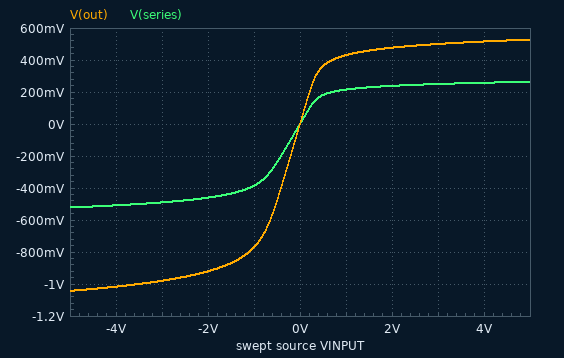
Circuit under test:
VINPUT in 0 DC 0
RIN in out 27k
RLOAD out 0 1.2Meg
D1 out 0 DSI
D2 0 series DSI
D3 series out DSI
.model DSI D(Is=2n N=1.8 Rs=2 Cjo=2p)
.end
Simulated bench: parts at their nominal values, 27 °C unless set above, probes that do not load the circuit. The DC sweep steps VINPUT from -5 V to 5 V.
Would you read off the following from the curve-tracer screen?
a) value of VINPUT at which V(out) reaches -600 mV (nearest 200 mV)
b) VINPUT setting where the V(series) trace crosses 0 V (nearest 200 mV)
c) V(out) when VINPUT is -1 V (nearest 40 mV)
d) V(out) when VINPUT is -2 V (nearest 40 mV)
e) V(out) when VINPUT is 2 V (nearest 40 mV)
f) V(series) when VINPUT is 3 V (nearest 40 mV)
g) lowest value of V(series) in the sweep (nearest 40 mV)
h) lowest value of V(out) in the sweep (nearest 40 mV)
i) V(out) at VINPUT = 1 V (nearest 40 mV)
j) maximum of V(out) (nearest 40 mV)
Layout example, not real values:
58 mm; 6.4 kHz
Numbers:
-600 mV; 0 V; -760 mV; -920 mV; 480 mV; 240 mV; -520 mV; -1.04 V; 440 mV; 520 mV
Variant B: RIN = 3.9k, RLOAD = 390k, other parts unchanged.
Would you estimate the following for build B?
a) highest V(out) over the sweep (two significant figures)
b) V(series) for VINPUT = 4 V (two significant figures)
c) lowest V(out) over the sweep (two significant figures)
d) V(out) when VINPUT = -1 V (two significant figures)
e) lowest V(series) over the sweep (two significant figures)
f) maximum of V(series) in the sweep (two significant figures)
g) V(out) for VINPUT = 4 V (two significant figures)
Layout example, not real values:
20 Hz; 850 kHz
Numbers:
620 mV; 300 mV; -1.2 V; -890 mV; -610 mV; 310 mV; 610 mV
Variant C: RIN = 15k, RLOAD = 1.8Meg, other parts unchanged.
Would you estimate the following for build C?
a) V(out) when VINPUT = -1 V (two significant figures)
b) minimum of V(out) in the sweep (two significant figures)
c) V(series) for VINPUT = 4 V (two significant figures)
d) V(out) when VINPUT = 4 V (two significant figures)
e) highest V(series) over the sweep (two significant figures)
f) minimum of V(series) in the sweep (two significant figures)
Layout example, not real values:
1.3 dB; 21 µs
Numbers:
-810 mV; -1.1 V; 270 mV; 540 mV; 280 mV; -550 mV
